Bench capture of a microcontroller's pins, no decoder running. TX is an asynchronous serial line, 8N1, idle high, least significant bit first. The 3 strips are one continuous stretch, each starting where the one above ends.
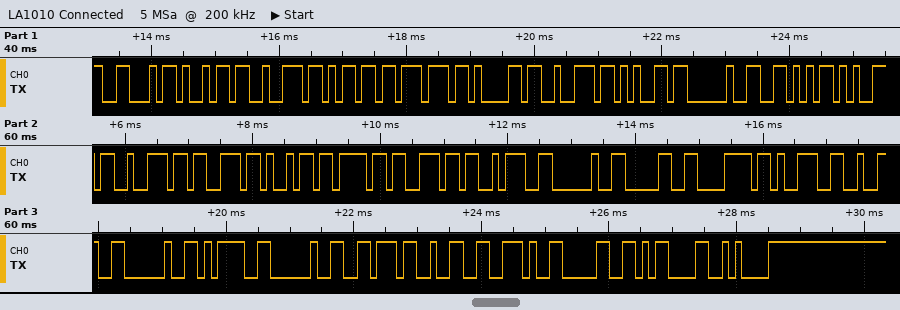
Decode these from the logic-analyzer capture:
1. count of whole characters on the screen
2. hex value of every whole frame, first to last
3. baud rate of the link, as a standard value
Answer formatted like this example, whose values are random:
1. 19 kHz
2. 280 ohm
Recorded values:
1. 31
2. 46 69 72 6D 77 61 72 65 20 56 65 72 73 69 6F 6E 3A 20 30 78 39 32 20 3D 20 76 32 2E 30 0D 0A
3. 9600 baud
